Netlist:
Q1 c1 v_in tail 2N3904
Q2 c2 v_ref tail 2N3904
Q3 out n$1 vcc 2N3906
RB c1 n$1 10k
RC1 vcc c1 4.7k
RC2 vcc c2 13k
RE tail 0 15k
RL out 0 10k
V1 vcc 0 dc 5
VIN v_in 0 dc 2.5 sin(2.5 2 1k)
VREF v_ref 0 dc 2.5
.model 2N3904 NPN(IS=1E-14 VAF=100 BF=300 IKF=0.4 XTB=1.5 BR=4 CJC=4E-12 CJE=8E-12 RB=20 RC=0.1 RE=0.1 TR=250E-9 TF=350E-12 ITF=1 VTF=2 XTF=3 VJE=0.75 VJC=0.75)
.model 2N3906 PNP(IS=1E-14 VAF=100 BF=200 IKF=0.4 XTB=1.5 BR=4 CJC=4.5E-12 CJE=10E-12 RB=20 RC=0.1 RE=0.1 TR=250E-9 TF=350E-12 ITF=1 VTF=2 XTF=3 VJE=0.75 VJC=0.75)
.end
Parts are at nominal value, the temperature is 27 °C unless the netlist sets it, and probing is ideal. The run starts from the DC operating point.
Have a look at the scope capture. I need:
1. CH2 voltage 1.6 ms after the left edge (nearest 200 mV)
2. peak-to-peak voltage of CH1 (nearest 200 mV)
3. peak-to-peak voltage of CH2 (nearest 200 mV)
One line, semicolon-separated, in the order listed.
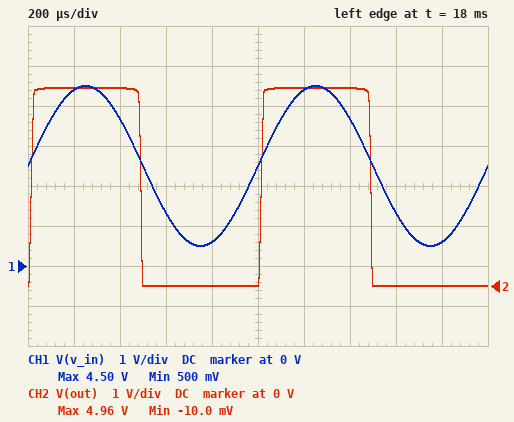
0 V; 4.0 V; 5.0 V
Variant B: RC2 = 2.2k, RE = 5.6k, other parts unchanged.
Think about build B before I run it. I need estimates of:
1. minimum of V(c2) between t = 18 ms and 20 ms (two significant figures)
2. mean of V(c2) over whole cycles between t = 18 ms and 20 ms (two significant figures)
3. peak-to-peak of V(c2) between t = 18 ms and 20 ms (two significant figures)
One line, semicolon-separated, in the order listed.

4.3 V; 4.6 V; 730 mV
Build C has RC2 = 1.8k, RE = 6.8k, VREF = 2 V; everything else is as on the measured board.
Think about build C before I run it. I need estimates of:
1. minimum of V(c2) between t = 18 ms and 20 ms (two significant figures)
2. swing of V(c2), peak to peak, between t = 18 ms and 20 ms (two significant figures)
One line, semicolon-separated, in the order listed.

4.6 V; 370 mV
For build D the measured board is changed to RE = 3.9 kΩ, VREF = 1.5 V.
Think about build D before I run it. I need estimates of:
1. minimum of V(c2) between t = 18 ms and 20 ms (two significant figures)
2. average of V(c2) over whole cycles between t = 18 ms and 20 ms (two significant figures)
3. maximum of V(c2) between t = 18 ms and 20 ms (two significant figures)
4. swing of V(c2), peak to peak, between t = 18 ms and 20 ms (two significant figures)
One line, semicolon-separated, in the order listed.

2.1 V; 4.0 V; 5.0 V; 2.9 V
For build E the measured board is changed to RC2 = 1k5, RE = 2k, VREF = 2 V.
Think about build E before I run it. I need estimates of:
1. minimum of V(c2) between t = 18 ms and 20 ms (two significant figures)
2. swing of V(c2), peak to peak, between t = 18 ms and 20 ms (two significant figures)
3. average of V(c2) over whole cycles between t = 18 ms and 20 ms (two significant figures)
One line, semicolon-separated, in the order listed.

4.0 V; 1.0 V; 4.6 V
